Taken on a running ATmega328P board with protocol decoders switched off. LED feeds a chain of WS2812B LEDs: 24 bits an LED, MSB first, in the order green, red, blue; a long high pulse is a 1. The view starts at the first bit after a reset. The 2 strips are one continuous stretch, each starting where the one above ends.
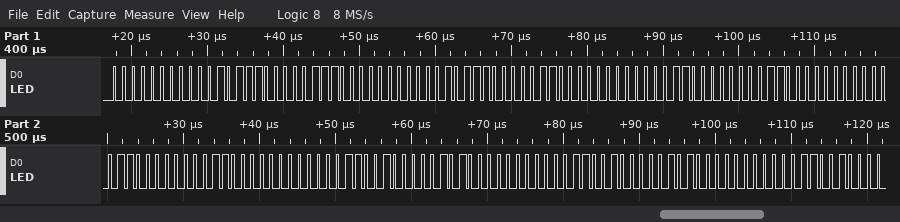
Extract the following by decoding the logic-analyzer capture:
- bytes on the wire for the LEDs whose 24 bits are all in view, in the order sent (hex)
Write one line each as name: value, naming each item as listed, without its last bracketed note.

bytes on the wire for the LEDs whose 24 bits are all in view, in the order sent: 00 17 07 00 17 06 00 18 06 00 18 06 00 19 05 00 19 05
